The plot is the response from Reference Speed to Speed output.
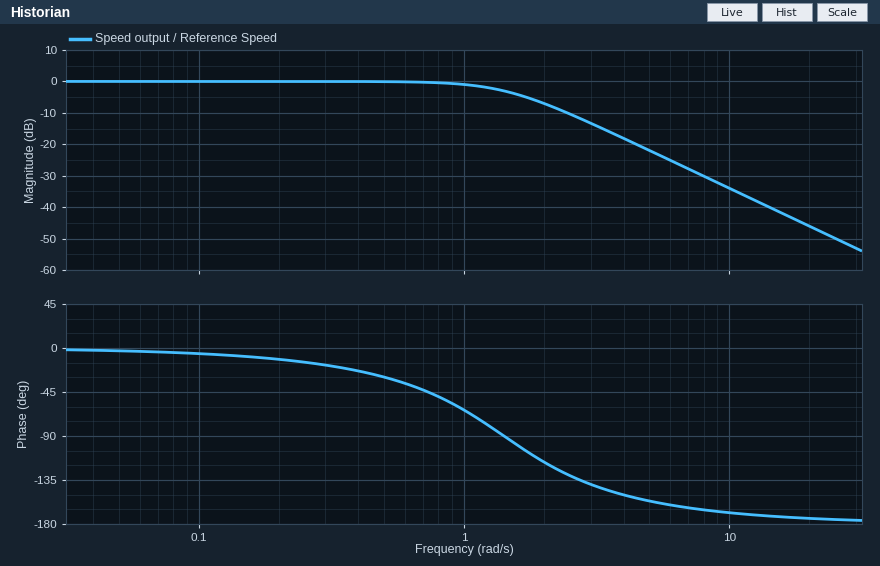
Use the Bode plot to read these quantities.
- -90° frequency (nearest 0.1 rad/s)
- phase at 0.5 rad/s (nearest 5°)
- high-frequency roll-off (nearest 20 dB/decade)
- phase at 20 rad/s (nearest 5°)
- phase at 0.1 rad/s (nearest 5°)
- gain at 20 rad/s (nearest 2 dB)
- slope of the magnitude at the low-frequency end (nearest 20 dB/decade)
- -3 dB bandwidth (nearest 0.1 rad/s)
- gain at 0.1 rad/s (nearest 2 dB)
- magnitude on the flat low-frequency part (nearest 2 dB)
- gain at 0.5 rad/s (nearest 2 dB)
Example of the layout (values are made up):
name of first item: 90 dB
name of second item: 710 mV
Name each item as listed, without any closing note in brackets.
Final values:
-90° frequency: 1.4 rad/s
phase at 0.5 rad/s: -30°
high-frequency roll-off: -40 dB/decade
phase at 20 rad/s: -175°
phase at 0.1 rad/s: -5°
gain at 20 rad/s: -46 dB
slope of the magnitude at the low-frequency end: 0 dB/decade
-3 dB bandwidth: 1.4 rad/s
gain at 0.1 rad/s: 0 dB
magnitude on the flat low-frequency part: 0 dB
gain at 0.5 rad/s: 0 dB
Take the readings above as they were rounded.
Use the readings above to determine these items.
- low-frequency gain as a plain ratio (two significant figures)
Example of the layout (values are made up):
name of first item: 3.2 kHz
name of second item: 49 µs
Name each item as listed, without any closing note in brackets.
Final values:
low-frequency gain as a plain ratio: 1.0
